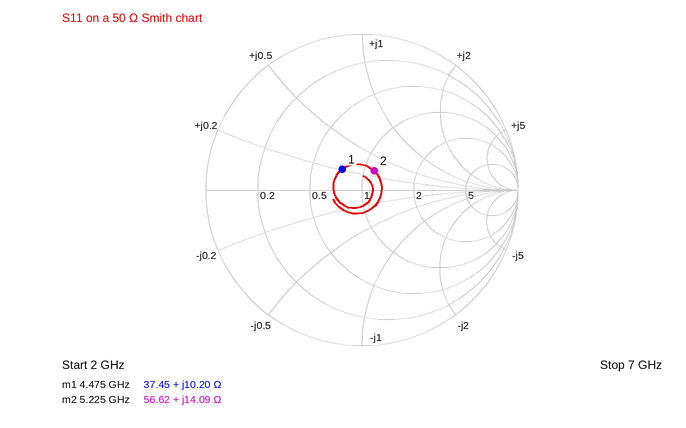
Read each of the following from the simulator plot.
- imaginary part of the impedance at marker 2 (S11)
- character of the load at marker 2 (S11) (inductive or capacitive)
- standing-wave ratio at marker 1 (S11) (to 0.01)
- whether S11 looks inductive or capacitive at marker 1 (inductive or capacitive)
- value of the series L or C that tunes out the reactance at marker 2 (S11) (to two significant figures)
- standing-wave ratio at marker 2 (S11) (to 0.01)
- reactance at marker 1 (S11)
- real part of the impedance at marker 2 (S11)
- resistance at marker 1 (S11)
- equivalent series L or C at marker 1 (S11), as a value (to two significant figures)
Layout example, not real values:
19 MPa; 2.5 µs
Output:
+14.09 Ω; inductive; 1.45; inductive; 2.2 pF; 1.34; +10.20 Ω; 56.62 Ω; 37.45 Ω; 360 pH
